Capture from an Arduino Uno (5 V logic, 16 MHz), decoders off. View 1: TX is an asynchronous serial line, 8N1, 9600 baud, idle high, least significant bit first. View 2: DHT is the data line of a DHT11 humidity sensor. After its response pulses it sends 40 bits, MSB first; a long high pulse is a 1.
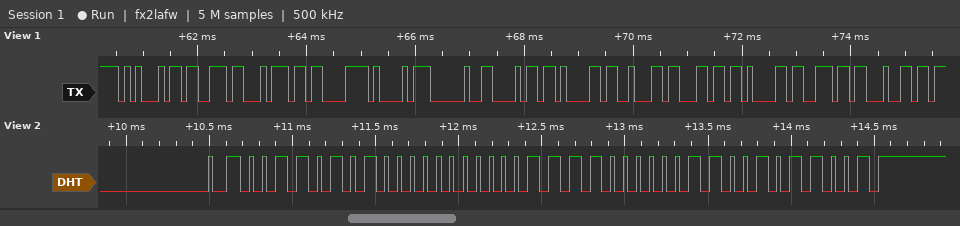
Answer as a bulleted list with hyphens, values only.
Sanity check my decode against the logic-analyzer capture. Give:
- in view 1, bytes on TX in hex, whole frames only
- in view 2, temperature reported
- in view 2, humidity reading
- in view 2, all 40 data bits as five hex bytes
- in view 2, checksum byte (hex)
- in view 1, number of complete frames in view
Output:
- 45 73 74 C3 A1 20 68 61 62 6C 61 6E 64
- 30.6 °C
- 53 %
- 35 00 1E 06 59
- 0x59
- 13
